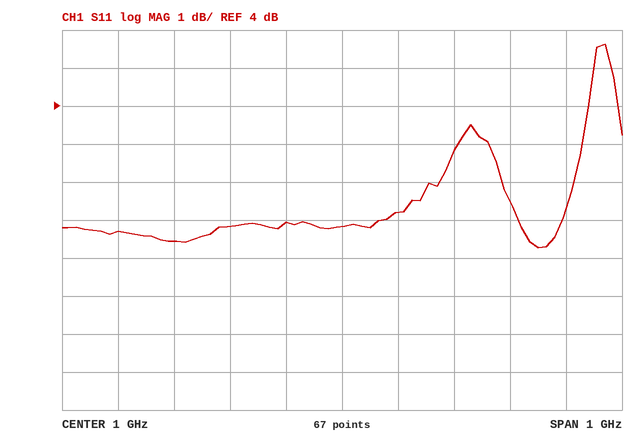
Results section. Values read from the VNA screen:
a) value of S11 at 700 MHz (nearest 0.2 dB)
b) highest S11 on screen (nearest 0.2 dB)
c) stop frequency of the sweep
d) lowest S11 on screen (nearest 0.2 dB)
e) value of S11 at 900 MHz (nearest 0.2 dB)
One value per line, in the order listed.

0.4 dB
5.6 dB
1.5 GHz
0.2 dB
1.0 dB
